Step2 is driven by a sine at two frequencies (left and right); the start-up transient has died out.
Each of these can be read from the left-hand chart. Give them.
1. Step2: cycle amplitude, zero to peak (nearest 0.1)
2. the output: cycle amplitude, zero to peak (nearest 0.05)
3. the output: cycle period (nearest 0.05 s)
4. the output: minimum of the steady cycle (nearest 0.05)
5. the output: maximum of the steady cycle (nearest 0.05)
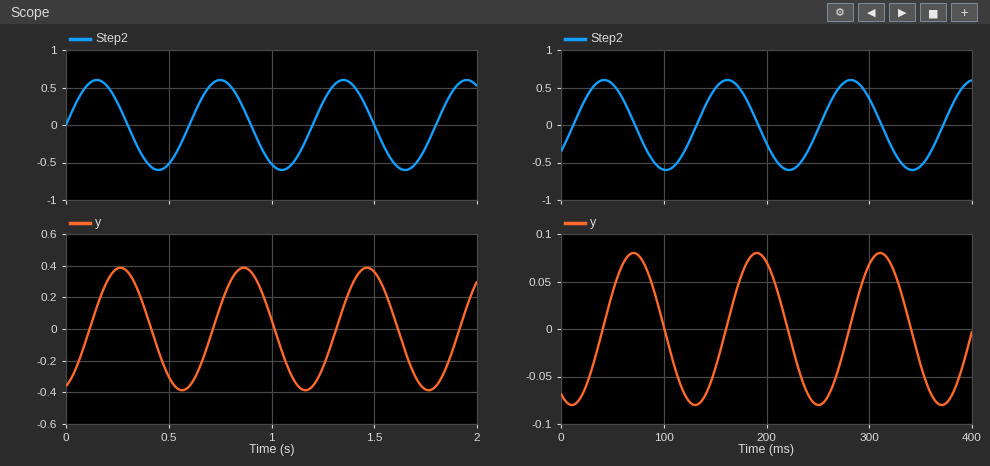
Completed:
0.6
0.40
0.60 s
-0.40
0.40
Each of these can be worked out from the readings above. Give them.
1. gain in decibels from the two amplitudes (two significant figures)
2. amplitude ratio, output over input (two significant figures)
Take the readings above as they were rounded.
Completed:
-3.5 dB
0.67
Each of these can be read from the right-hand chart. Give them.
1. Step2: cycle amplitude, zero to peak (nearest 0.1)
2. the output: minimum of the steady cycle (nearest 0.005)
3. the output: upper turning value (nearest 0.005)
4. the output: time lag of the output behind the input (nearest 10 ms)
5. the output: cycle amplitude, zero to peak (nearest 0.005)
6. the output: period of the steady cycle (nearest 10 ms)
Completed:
0.6
-0.080
0.080
30 ms
0.080
120 ms
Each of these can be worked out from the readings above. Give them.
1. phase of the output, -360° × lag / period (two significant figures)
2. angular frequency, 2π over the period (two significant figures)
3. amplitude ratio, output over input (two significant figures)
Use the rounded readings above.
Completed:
-90°
0.052 rad/ms
0.13
